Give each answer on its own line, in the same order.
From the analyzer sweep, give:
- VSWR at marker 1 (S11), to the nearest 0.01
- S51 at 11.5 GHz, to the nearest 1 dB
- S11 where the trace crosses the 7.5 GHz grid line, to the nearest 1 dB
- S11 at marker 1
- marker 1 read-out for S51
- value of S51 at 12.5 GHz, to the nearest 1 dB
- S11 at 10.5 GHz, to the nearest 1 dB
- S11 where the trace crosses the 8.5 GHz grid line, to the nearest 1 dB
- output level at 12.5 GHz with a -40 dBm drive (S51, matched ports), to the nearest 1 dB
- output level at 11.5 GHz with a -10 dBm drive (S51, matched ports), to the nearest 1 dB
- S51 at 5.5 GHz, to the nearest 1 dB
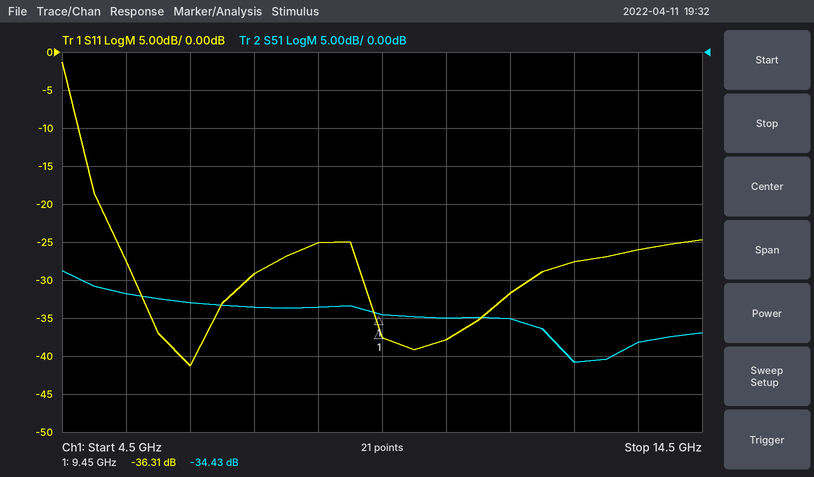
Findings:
1.03
-35 dB
-29 dB
-36.31 dB
-34.43 dB
-41 dB
-38 dB
-25 dB
-81 dBm
-45 dBm
-32 dB
